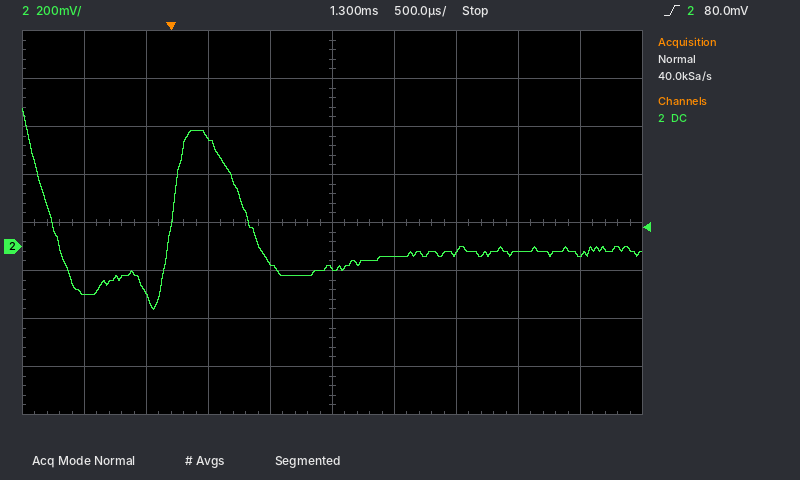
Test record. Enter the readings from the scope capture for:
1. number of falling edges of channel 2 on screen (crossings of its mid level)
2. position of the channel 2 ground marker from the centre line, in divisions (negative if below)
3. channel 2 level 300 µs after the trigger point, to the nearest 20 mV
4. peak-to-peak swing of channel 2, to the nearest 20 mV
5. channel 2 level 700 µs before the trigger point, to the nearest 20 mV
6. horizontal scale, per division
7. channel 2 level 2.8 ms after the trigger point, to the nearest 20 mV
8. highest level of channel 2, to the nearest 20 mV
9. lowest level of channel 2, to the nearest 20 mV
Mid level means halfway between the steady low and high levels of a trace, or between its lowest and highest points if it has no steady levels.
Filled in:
2
-0.5 div
460 mV
840 mV
-200 mV
500 µs
-20 mV
580 mV
-260 mV
